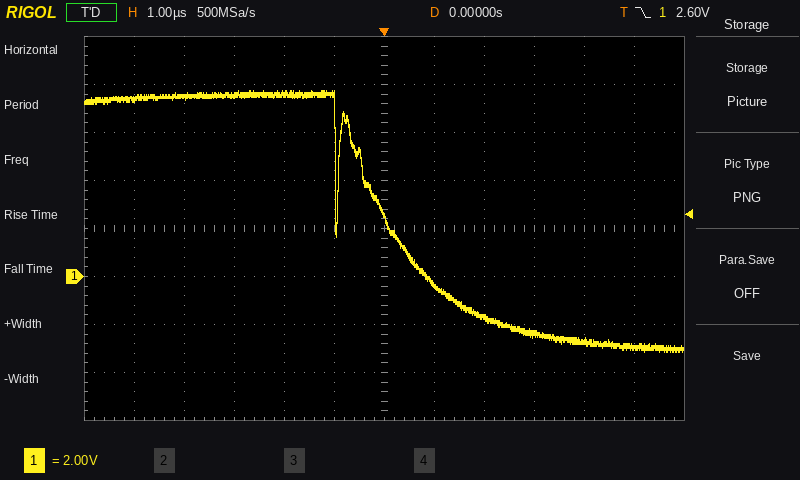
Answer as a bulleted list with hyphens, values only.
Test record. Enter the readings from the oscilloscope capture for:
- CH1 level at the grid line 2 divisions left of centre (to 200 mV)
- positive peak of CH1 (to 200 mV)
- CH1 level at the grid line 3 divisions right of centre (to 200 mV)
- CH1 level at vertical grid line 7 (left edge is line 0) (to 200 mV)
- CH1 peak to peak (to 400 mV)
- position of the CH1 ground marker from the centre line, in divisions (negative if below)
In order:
- 7.6 V
- 7.8 V
- -2.4 V
- -400 mV
- 10.8 V
- -1.0 div
